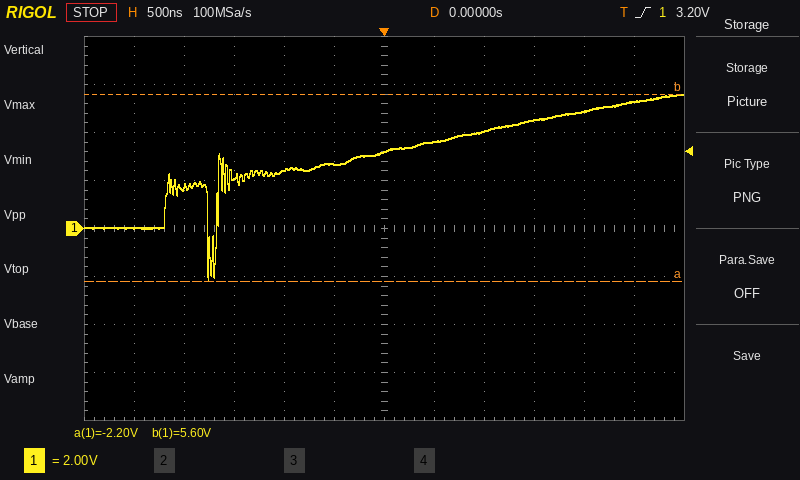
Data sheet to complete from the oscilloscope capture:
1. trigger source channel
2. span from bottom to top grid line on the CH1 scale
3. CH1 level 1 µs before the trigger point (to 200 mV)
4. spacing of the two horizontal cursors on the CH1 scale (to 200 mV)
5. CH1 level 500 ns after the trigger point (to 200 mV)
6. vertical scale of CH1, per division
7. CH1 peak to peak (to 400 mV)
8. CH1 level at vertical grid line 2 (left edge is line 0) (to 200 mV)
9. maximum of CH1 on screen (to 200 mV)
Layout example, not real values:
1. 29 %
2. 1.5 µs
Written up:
1. CH1
2. 16 V
3. 2.4 V
4. 7.8 V
5. 3.6 V
6. 2 V
7. 7.6 V
8. 1.8 V
9. 5.6 V
